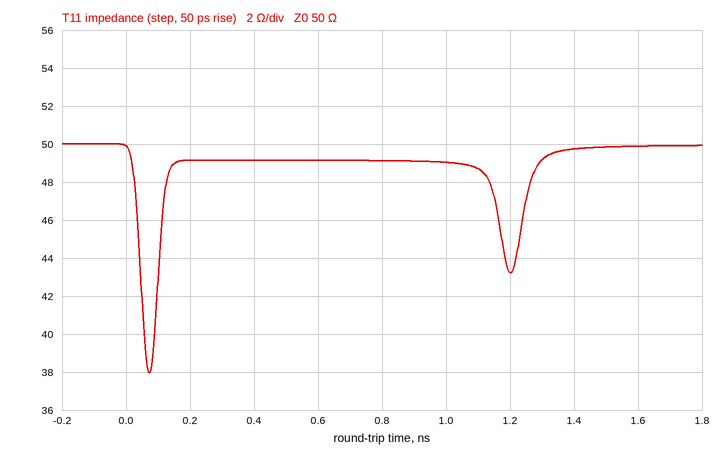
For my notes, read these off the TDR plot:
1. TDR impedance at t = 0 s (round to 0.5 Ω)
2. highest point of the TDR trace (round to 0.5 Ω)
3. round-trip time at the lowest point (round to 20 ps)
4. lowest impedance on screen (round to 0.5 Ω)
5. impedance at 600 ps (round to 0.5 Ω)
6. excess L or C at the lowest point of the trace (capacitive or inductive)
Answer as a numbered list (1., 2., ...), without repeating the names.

1. 50.0 Ω
2. 50.0 Ω
3. 80 ps
4. 38.0 Ω
5. 49.0 Ω
6. capacitive
